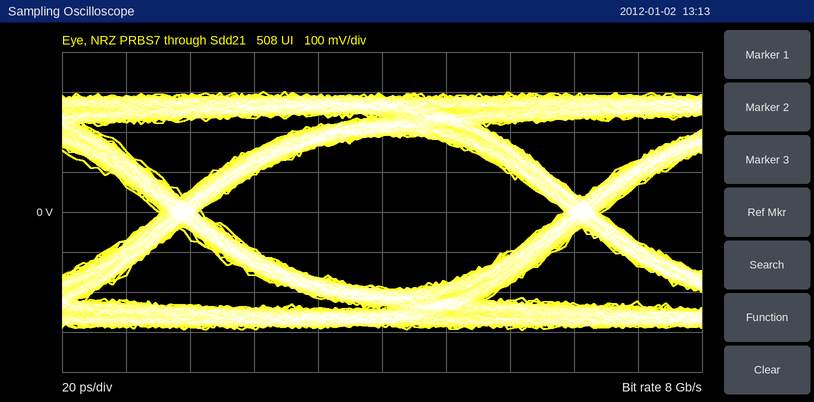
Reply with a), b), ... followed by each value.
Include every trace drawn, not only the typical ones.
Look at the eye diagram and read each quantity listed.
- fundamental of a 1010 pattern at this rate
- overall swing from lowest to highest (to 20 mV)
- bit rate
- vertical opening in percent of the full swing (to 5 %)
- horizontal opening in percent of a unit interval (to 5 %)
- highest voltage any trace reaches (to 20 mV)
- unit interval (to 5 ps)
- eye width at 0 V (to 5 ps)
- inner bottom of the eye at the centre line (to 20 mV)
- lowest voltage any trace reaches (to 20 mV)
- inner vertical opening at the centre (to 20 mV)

a) 4 GHz
b) 600 mV
c) 8 Gb/s
d) 65 %
e) 90 %
f) 300 mV
g) 125 ps
h) 115 ps
i) -180 mV
j) -300 mV
k) 380 mV
